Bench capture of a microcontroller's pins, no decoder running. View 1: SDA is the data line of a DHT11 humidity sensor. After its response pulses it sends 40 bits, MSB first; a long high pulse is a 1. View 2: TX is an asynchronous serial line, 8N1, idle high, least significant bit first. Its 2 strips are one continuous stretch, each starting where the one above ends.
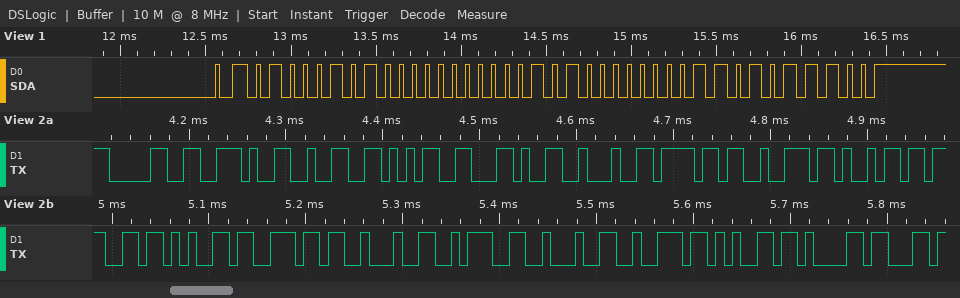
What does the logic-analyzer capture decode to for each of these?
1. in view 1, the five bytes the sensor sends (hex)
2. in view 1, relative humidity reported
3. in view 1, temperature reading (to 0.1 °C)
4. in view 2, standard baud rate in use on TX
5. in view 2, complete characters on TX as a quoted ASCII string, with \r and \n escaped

45 00 14 03 5C
69 %
20.3 °C
115200 baud
"0.25,\"origen\":\"rea"
